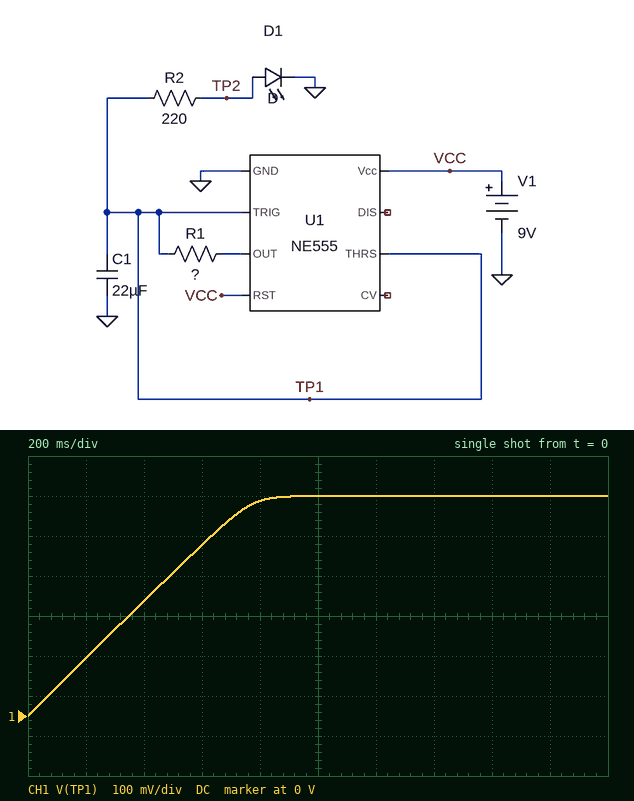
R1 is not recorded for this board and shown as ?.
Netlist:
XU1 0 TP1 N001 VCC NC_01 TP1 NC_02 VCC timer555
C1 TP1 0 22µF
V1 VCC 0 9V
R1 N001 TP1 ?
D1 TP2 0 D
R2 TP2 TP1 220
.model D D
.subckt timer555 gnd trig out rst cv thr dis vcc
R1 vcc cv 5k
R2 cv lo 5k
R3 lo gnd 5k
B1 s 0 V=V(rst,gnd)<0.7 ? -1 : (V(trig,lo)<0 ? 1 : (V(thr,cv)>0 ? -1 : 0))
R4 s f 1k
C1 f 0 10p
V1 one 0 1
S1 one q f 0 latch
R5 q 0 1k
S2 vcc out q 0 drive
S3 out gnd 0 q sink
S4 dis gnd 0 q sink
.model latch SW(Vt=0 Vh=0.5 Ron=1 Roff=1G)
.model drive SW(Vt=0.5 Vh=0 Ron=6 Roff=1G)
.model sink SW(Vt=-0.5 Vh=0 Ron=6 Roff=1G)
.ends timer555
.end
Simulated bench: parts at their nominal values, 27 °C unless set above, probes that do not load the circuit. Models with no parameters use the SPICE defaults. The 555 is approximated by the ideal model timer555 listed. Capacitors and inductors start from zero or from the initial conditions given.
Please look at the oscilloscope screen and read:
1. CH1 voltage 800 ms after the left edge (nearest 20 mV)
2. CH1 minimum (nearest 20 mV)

540 mV
0 V
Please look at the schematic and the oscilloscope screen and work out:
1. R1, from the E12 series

560 kΩ
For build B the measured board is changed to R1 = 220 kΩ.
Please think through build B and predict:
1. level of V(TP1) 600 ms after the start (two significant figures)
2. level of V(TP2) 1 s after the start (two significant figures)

580 mV
570 mV
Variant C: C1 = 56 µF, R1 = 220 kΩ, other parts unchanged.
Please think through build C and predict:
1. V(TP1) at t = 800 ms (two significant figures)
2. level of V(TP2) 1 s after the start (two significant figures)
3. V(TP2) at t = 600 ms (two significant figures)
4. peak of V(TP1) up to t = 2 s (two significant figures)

550 mV
570 mV
430 mV
580 mV
